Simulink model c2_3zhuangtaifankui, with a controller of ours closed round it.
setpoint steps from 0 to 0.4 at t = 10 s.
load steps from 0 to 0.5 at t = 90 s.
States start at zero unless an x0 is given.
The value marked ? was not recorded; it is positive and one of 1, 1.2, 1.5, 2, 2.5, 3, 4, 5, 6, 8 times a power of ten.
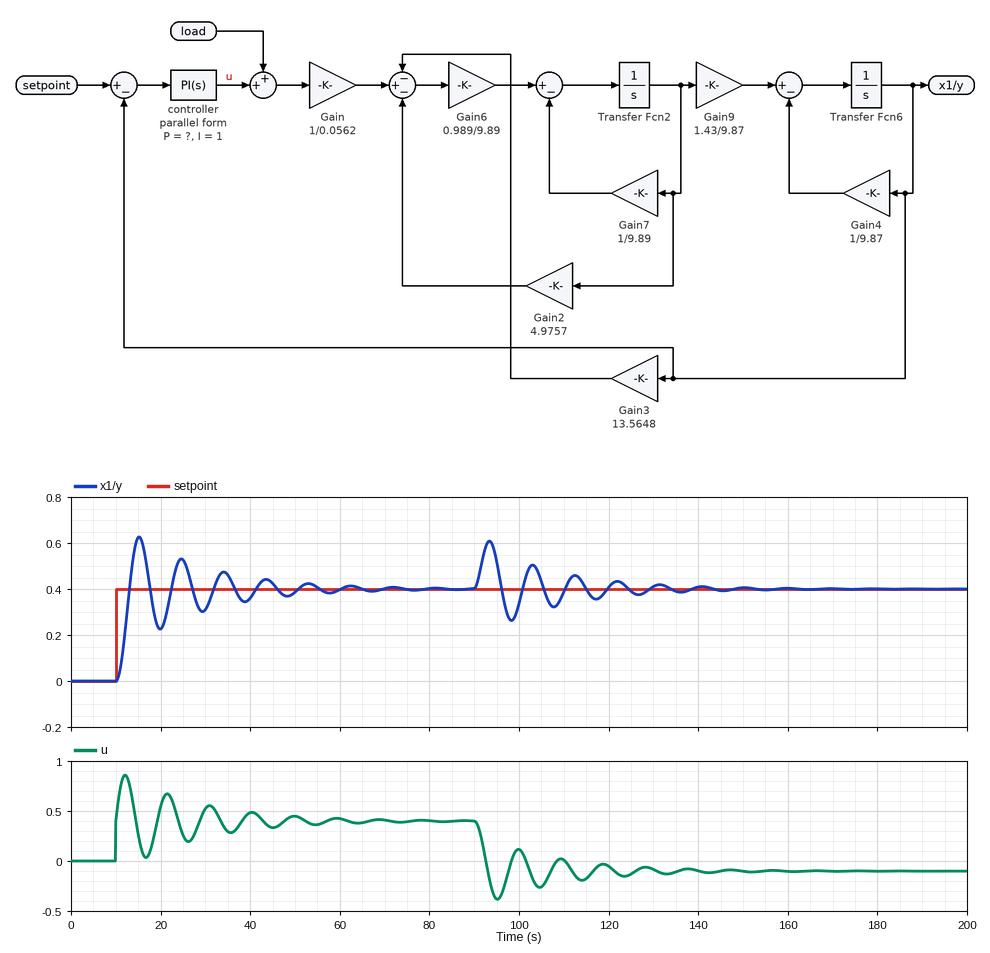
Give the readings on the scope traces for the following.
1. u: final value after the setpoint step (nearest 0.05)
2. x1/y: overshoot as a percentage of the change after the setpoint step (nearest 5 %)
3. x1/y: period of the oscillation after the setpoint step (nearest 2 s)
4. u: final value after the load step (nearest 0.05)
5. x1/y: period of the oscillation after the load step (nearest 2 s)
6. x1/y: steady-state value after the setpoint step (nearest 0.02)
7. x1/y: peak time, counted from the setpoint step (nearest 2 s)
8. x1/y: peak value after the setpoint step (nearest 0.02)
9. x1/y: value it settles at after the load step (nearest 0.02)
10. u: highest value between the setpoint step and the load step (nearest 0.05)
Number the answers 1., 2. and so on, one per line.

1. 0.40
2. 55 %
3. 10 s
4. -0.10
5. 10 s
6. 0.40
7. 6 s
8. 0.62
9. 0.40
10. 0.85
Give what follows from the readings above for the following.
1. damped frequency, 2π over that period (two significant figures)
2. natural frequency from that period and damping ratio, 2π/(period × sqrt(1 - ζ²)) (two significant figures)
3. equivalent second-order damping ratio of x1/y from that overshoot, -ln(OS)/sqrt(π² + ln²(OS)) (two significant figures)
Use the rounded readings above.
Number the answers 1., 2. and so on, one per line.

1. 0.63 rad/s
2. 0.64 rad/s
3. 0.19
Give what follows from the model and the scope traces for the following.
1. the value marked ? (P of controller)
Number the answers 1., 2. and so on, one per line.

1. 1
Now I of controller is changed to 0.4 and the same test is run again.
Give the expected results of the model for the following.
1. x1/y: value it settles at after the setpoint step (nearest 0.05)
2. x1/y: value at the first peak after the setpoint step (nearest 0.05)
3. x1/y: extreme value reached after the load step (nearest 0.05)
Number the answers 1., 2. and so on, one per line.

1. 0.40
2. 0.45
3. 0.65
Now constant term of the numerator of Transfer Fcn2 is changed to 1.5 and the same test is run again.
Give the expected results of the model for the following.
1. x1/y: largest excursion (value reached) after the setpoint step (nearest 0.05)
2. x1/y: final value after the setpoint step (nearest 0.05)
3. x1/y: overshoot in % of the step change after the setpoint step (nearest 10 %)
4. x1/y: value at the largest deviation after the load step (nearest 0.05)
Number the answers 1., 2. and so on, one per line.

1. 0.55
2. 0.40
3. 40 %
4. 0.60
